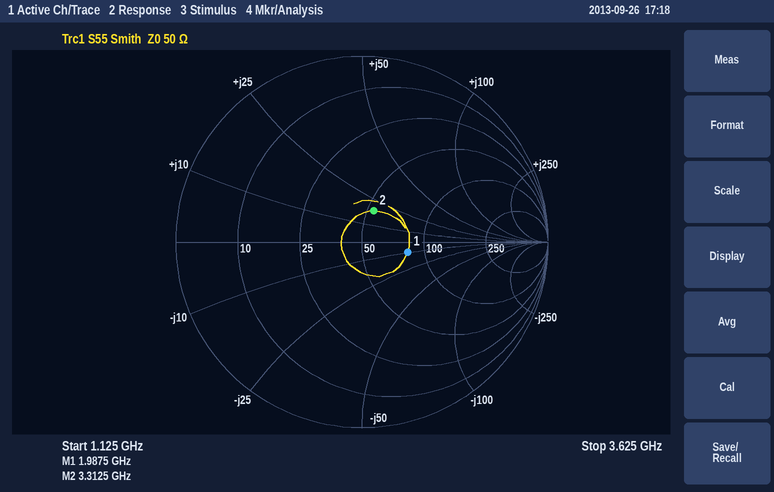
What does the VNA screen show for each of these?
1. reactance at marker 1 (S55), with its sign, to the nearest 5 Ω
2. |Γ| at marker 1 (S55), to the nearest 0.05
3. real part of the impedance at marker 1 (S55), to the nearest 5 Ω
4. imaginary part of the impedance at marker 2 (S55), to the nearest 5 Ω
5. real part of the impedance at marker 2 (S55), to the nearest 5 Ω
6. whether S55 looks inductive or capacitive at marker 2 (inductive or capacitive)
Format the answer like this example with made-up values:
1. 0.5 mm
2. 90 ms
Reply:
1. -10 Ω
2. 0.25
3. 80 Ω
4. +20 Ω
5. 55 Ω
6. inductive
